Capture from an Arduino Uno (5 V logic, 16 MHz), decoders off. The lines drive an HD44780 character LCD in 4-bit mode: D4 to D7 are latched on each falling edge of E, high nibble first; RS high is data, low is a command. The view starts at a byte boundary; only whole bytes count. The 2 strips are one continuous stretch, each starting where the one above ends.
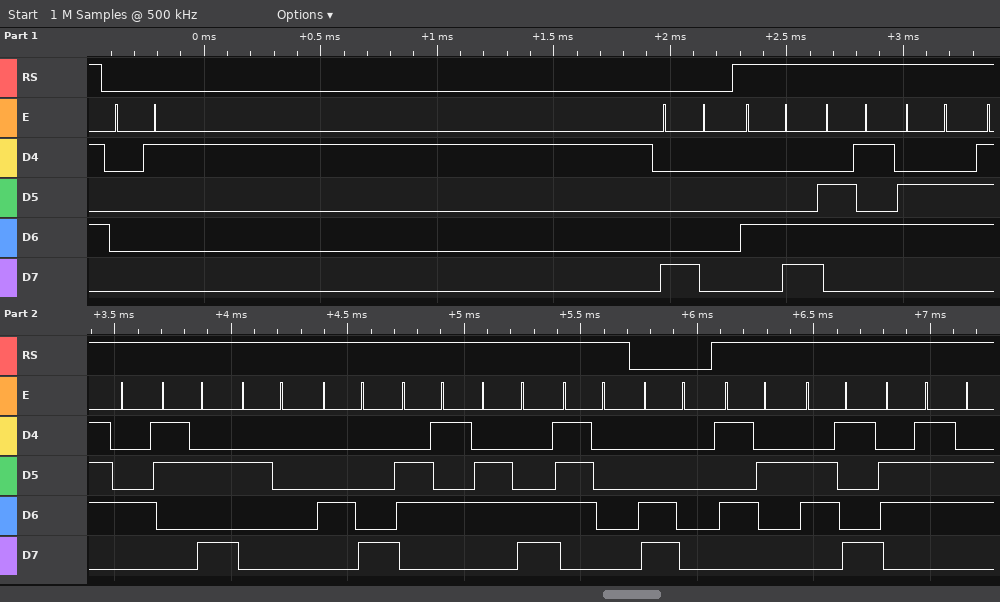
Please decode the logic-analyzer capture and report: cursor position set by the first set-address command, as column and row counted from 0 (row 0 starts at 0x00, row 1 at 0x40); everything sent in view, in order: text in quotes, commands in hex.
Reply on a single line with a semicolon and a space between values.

column 0, row 0; 0x01 0x80 "Left: Help" 0xC0 "Rig"
